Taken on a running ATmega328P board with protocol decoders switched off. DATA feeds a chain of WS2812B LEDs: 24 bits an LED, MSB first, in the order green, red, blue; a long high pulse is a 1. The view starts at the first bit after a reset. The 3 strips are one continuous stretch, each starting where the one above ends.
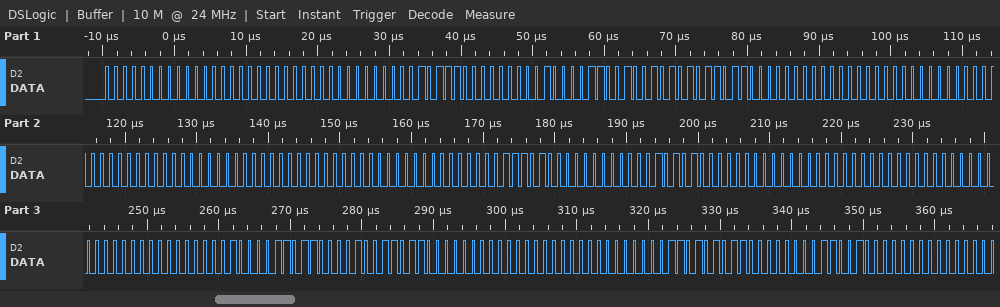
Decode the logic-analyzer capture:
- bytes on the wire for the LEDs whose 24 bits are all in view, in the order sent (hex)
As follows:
00 00 00 00 17 00 43 25 5B 00 00 00 00 00 00 00 00 00 3A 00 15 00 00 00 00 00 00 43 61 36 00 00 00 35 60 19
